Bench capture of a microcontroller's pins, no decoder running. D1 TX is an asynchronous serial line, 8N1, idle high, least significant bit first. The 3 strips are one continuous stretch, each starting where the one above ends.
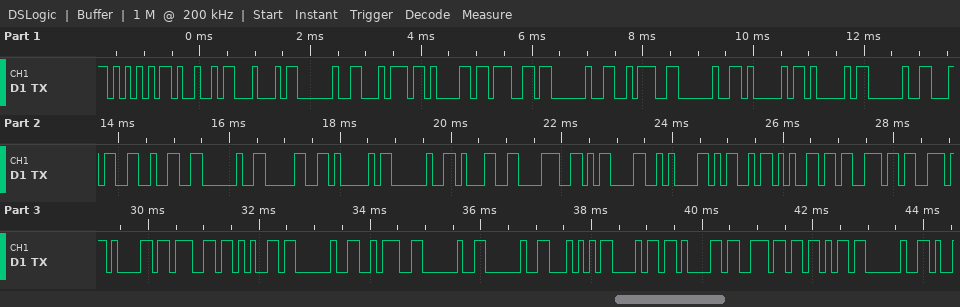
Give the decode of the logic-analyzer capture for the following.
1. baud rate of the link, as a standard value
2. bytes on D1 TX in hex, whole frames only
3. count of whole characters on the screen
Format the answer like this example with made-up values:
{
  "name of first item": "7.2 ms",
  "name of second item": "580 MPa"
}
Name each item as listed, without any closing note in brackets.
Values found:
{
  "baud rate of the link, as a standard value": "9600 baud",
  "bytes on D1 TX in hex, whole frames only": "55 49 44 20 74 61 67 20 3A 20 41 41 20 34 32 20 30 41 20 31 38 0D 0A 4D 65 73 73 61 67 65 20 3A 20 20 54 68 61 6E 6B 20",
  "count of whole characters on the screen": "40"
}
